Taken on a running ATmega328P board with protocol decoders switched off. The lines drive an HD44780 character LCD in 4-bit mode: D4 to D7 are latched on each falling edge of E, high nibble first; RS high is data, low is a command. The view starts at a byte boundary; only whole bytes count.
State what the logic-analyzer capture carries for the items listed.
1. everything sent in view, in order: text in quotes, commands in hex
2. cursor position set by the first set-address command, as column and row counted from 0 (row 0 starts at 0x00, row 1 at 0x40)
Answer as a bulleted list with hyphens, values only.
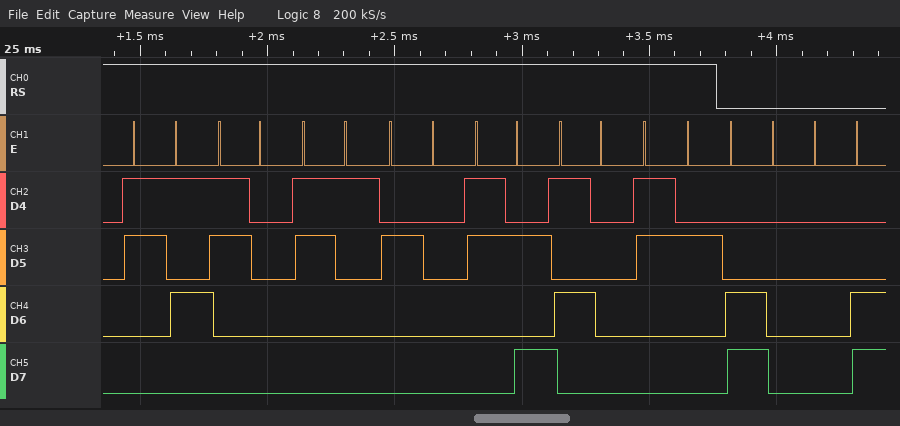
- "501 :P2" 0xC0 0x0C
- column 0, row 1
